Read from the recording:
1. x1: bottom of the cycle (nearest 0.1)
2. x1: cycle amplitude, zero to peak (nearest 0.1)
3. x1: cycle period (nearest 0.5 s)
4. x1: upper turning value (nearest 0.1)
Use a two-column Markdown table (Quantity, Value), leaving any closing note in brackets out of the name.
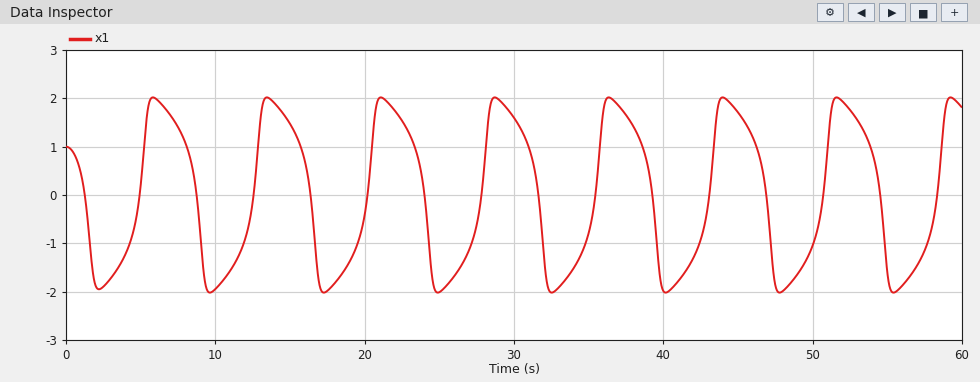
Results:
| Quantity | Value |
|---|---|
| x1: bottom of the cycle | -2.0 |
| x1: cycle amplitude, zero to peak | 2.0 |
| x1: cycle period | 7.5 s |
| x1: upper turning value | 2.0 |
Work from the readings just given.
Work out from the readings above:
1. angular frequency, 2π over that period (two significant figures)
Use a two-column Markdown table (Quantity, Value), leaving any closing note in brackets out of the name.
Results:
| Quantity | Value |
|---|---|
| angular frequency, 2π over that period | 0.84 rad/s |
